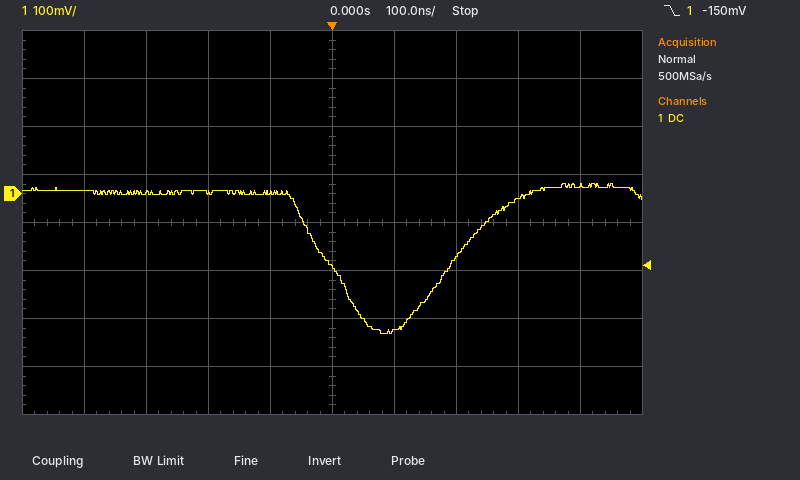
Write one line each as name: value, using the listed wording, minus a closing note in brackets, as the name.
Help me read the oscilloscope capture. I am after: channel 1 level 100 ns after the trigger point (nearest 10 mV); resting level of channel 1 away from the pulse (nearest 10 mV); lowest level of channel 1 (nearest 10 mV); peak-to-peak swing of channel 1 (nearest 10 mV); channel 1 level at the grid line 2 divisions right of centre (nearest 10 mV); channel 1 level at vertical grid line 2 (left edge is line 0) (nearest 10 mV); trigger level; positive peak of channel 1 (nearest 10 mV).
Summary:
channel 1 level 100 ns after the trigger point: -290 mV
resting level of channel 1 away from the pulse: 0 mV
lowest level of channel 1: -290 mV
peak-to-peak swing of channel 1: 310 mV
channel 1 level at the grid line 2 divisions right of centre: -130 mV
channel 1 level at vertical grid line 2 (left edge is line 0): 0 mV
trigger level: -150 mV
positive peak of channel 1: 20 mV
